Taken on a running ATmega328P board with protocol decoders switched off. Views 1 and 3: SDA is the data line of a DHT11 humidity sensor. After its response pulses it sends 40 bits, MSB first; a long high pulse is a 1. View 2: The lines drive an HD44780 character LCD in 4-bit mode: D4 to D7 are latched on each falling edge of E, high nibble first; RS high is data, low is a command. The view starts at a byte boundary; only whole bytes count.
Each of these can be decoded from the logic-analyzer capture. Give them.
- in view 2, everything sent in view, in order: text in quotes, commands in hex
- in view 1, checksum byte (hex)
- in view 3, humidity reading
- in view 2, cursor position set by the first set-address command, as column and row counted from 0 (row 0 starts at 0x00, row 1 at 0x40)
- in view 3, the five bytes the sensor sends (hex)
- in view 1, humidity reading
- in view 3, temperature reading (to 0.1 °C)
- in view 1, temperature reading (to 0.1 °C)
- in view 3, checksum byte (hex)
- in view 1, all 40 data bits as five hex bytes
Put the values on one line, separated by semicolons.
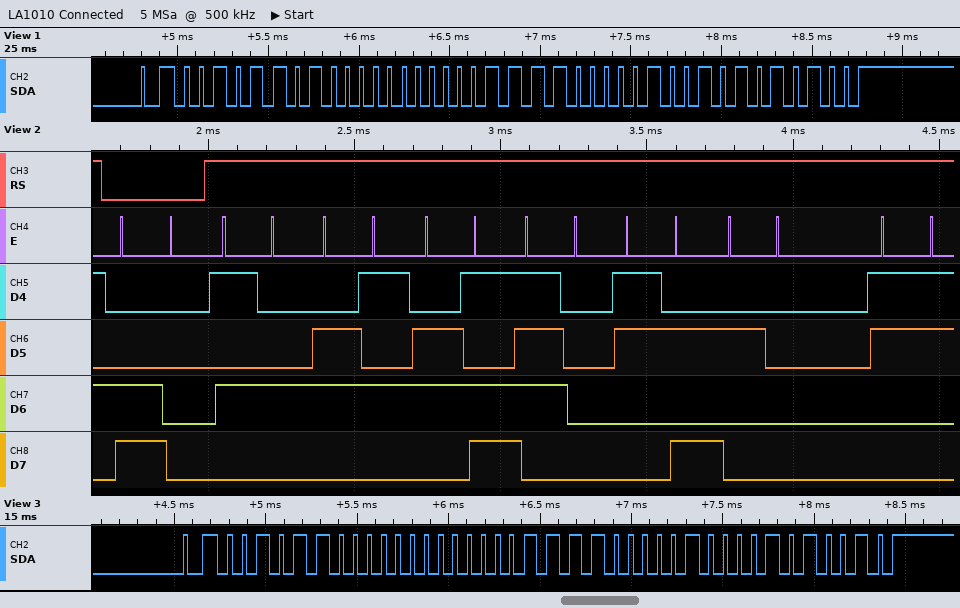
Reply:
0xC0 "Temp: 3"; 0x54; 44 %; column 0, row 1; 2C 00 1E 08 52; 45 %; 30.8 °C; 30.9 °C; 0x52; 2D 00 1E 09 54
